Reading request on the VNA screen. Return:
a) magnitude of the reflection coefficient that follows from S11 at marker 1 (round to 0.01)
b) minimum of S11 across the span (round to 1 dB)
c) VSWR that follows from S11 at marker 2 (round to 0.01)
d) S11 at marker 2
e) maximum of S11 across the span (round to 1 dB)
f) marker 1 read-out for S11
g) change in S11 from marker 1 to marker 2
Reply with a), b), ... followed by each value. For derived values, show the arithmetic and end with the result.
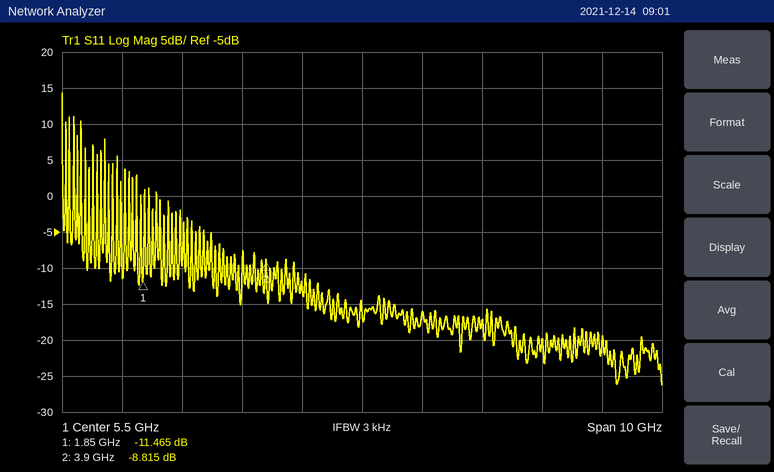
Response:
a) 10^(-11.465/20) ≈ 0.27
b) -26 dB
c) (1 + 0.3625)/(1 − 0.3625) ≈ 2.14
d) -8.815 dB
e) 14 dB
f) -11.465 dB
g) -8.815 − (-11.465) = 2.650 dB
